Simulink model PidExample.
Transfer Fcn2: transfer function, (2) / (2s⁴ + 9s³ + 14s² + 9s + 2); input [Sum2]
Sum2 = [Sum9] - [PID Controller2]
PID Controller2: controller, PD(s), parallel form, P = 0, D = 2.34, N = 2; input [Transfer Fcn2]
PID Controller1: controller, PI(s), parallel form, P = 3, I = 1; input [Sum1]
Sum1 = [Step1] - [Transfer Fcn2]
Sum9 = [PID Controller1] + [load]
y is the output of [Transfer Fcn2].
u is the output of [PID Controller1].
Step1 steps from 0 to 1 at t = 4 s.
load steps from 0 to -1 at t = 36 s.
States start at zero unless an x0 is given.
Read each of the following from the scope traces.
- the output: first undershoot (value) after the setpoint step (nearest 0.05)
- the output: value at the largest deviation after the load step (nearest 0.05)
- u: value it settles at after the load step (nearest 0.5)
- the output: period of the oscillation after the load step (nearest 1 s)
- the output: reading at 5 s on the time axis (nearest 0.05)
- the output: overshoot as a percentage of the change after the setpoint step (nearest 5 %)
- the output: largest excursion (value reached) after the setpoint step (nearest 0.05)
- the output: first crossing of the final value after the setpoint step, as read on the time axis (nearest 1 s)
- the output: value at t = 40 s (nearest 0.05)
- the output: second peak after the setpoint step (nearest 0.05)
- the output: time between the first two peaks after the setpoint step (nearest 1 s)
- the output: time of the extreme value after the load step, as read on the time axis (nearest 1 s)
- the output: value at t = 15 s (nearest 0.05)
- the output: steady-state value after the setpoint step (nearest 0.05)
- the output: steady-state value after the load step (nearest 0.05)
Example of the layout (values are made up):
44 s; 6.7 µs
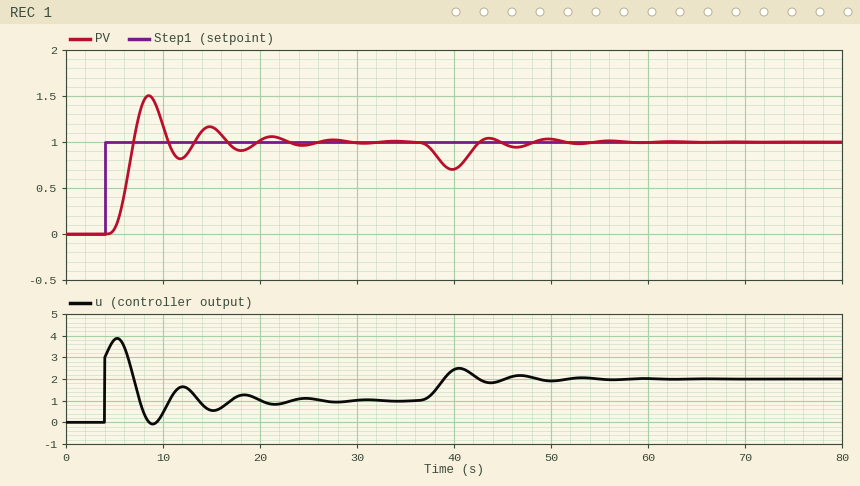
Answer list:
0.80; 0.70; 2.0; 7 s; 0.05; 50 %; 1.50; 7 s; 0.70; 1.15; 6 s; 40 s; 1.15; 1.00; 1.00
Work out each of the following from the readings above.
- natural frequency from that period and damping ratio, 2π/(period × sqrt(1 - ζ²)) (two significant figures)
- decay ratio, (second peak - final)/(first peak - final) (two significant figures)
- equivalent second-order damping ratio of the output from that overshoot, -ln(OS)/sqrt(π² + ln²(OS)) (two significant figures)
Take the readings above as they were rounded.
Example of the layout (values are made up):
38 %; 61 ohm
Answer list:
1.1 rad/s; 0.30; 0.22
